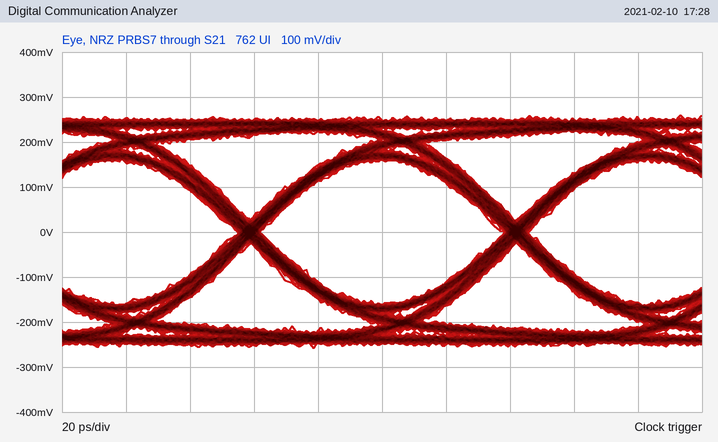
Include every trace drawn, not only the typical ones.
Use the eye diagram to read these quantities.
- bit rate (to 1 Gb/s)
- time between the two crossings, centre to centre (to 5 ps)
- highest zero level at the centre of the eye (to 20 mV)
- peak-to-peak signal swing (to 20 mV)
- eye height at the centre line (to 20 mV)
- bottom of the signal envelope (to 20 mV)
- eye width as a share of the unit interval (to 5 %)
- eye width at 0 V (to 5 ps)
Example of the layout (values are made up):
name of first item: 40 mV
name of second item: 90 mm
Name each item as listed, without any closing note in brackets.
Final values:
bit rate: 12 Gb/s
time between the two crossings, centre to centre: 85 ps
highest zero level at the centre of the eye: -160 mV
peak-to-peak signal swing: 520 mV
eye height at the centre line: 320 mV
bottom of the signal envelope: -260 mV
eye width as a share of the unit interval: 90 %
eye width at 0 V: 75 ps
